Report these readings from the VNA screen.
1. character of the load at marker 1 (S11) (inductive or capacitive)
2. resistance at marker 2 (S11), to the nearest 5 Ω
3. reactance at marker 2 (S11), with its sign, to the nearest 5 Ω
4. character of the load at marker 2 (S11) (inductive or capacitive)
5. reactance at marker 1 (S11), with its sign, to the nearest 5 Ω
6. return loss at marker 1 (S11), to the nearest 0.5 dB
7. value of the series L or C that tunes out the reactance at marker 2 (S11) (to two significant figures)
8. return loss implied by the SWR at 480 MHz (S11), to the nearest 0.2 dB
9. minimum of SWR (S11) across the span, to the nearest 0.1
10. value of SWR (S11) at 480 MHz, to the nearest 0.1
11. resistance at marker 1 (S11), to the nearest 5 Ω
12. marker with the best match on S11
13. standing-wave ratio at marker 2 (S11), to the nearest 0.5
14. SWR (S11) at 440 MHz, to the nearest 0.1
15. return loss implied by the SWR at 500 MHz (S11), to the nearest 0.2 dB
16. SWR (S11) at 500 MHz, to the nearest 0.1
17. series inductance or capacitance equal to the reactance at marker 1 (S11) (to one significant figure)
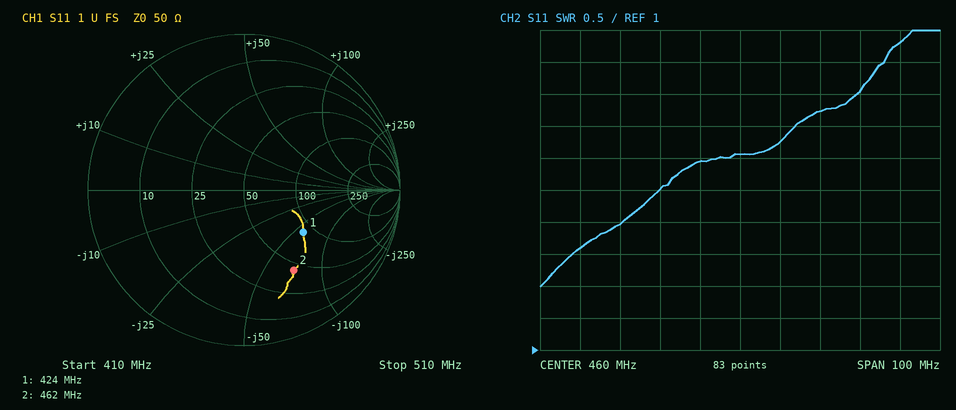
capacitive
45 Ω
-70 Ω
capacitive
-60 Ω
6.5 dB
24 nH
3.8 dB
2.0
4.7
85 Ω
marker 1
4.0
3.5
3.0 dB
5.8
6 pF
